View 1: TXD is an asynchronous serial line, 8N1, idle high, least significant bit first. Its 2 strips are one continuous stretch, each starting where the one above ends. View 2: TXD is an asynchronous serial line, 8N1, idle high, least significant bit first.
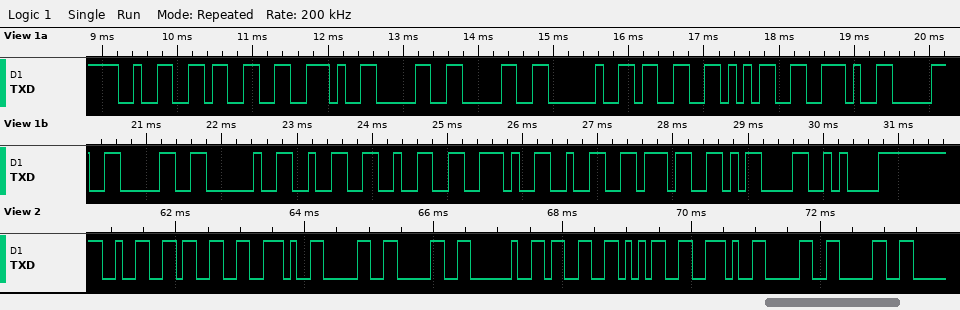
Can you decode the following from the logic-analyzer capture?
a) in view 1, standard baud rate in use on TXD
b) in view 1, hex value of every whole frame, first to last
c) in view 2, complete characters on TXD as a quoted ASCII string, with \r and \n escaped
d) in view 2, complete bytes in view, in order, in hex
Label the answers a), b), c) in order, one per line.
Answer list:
a) 9600 baud
b) 32 33 2E 30 30 20 33 35 2E 30 30 20 32 32 2E 32 37 0D 0A
c) "23.00 35.00"
d) 32 33 2E 30 30 20 33 35 2E 30 30
